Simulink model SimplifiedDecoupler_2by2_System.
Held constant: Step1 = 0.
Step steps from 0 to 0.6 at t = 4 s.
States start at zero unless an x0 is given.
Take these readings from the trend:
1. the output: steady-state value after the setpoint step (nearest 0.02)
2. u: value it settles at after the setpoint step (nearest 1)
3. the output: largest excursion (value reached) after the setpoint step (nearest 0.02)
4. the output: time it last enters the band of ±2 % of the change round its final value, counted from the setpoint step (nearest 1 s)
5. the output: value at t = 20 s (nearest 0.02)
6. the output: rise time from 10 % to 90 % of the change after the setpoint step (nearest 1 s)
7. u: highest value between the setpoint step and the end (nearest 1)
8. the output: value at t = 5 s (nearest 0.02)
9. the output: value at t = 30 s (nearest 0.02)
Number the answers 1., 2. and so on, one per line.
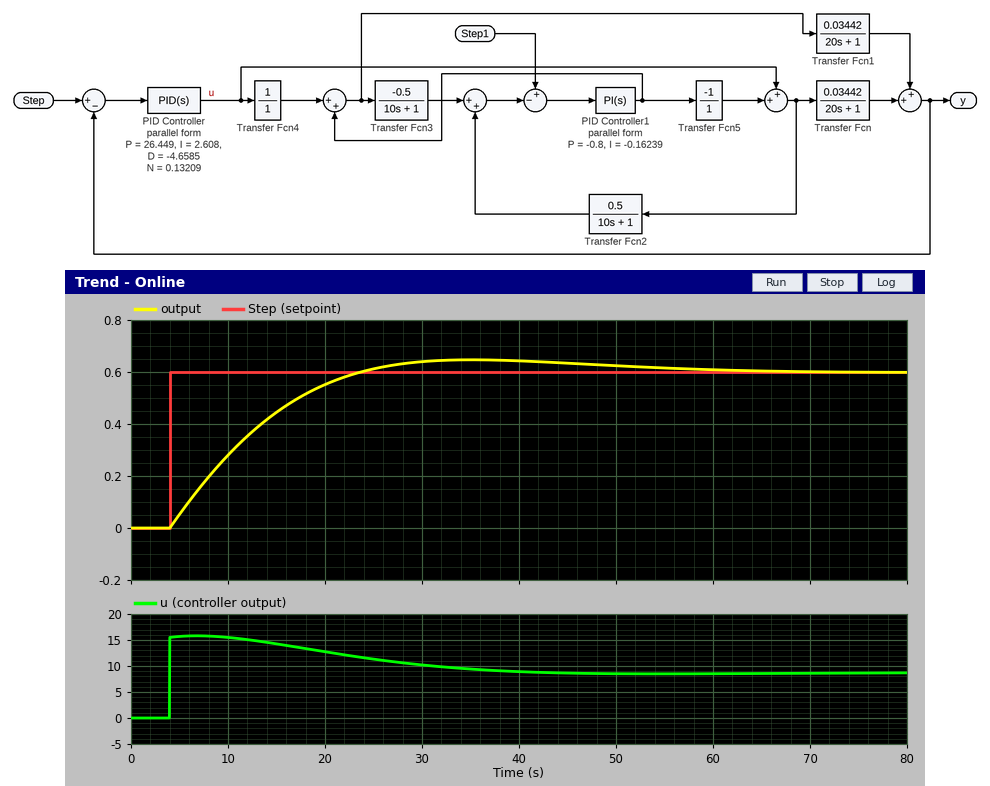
1. 0.60
2. 9
3. 0.64
4. 53 s
5. 0.56
6. 14 s
7. 16
8. 0.06
9. 0.64
